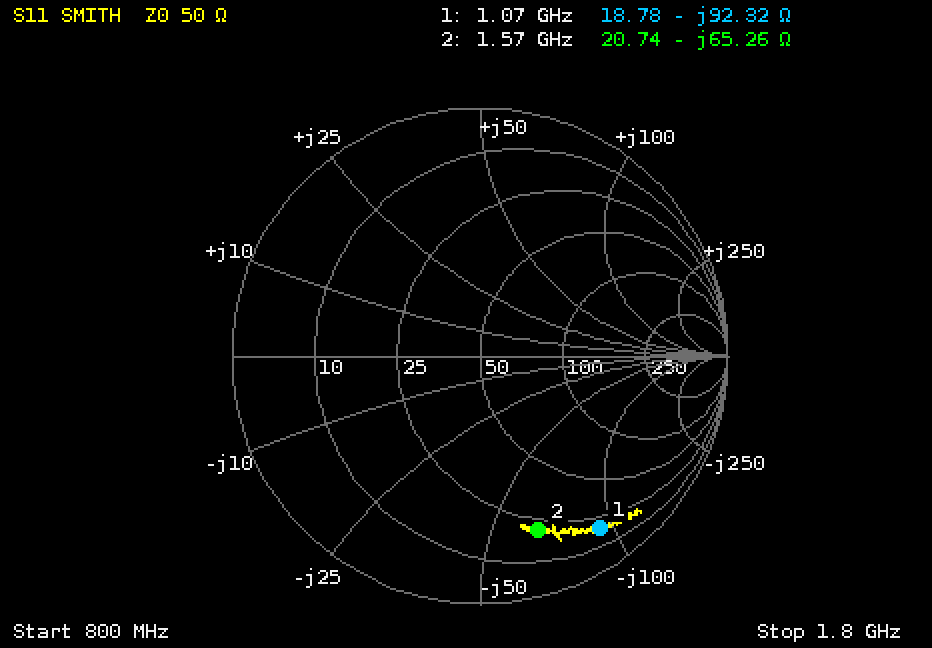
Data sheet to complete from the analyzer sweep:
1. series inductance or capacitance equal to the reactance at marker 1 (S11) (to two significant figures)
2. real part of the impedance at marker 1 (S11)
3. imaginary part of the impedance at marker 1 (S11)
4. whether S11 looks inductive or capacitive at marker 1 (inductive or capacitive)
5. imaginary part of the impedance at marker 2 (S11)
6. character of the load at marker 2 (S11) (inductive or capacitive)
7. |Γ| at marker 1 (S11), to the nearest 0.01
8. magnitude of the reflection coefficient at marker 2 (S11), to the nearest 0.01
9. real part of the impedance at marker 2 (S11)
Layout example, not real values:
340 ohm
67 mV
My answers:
1.6 pF
18.78 Ω
-92.32 Ω
capacitive
-65.26 Ω
capacitive
0.85
0.74
20.74 Ω
